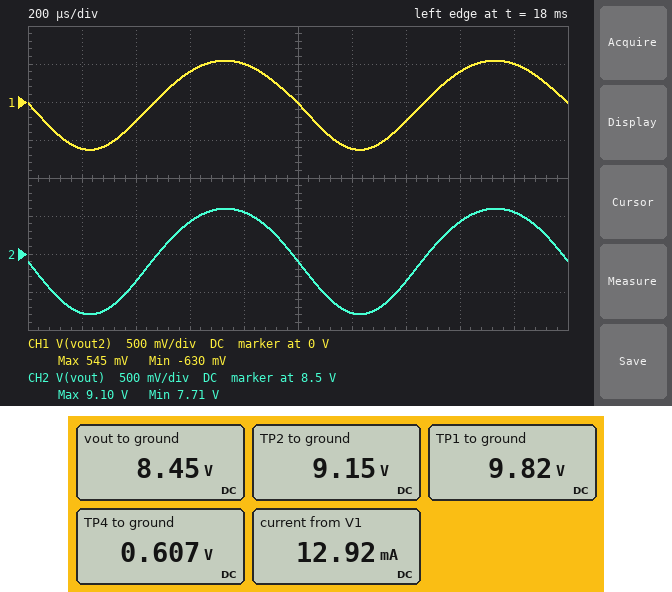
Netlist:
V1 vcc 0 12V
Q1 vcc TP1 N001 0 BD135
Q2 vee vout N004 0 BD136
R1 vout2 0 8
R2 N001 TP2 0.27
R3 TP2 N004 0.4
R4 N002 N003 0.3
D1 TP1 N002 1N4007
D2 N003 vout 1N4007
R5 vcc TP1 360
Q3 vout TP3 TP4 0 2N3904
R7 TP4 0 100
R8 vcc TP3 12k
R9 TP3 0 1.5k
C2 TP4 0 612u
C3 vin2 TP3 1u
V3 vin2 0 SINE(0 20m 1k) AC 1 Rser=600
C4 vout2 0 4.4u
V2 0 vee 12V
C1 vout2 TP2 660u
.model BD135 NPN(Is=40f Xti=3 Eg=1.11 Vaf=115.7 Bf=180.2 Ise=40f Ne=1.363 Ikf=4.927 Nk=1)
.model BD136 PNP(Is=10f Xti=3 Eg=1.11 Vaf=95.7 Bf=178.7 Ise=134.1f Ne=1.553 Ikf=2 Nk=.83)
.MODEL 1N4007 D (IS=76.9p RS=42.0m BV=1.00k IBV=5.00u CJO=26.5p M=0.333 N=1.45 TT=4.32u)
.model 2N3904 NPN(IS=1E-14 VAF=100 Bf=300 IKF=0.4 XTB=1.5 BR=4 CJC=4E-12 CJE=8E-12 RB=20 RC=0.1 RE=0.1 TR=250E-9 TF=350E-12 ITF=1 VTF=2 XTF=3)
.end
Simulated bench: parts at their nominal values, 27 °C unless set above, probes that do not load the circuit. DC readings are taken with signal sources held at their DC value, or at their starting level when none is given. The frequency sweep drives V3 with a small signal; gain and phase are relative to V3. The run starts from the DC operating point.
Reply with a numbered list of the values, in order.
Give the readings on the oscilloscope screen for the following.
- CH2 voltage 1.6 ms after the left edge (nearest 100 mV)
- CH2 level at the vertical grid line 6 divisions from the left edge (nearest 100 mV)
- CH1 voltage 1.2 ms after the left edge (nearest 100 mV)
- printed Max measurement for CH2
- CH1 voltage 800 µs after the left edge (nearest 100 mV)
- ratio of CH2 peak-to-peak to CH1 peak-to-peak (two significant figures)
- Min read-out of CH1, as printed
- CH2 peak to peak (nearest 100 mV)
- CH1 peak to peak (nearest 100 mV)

1. 8.9 V
2. 7.7 V
3. -600 mV
4. 9.10 V
5. 500 mV
6. 1.2
7. -630 mV
8. 1.4 V
9. 1.2 V
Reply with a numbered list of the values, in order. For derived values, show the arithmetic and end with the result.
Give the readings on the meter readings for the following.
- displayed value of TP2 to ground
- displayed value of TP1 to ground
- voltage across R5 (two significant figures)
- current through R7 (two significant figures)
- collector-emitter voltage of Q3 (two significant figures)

1. 9.15 V
2. 9.82 V
3. 12 V - 9.82 V = 2.2 V
4. (607 mV) / 100 Ω = 6.1 mA
5. 8.45 V - 607 mV = 7.8 V
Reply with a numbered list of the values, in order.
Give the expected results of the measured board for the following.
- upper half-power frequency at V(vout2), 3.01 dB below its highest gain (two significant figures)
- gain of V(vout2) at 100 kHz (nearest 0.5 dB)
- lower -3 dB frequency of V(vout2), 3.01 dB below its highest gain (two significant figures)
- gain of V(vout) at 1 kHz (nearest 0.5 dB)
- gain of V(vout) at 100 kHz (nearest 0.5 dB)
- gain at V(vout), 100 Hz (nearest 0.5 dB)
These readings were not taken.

1. 13 kHz
2. 11.0 dB
3. 150 Hz
4. 31.0 dB
5. 27.0 dB
6. 26.0 dB
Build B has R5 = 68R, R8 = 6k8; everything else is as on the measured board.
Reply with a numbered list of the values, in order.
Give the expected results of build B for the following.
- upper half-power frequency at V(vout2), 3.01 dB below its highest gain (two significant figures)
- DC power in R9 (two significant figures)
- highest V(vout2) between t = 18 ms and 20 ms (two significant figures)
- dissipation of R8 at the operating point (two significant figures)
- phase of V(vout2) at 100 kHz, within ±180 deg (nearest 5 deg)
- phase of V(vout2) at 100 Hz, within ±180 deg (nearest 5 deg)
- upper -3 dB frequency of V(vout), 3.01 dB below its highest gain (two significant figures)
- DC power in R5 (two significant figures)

1. 32 kHz
2. 3.0 mW
3. 220 mV
4. 14 mW
5. 105 deg
6. -85 deg
7. 120 kHz
8. 13 mW
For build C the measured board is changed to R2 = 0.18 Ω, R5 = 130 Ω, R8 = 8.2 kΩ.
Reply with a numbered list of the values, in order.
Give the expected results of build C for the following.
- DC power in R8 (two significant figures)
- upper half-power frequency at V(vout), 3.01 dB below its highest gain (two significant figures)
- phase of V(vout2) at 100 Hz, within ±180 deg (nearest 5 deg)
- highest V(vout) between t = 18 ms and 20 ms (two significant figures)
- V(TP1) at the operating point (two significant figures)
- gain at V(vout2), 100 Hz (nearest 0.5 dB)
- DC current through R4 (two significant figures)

1. 13 mW
2. 53 kHz
3. -90 deg
4. 9.6 V
5. 11 V
6. 18.5 dB
7. 11 mA
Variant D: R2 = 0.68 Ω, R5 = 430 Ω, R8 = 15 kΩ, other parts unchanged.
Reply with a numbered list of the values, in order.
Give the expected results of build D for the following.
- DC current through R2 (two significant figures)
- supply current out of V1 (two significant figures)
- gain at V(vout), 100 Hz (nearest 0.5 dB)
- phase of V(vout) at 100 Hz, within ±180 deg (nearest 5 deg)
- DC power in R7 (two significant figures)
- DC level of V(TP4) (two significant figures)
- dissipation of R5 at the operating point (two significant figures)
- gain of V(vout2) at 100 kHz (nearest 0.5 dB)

1. 3.1 mA
2. 7.7 mA
3. 26.0 dB
4. -120 deg
5. 1.5 mW
6. 390 mV
7. 6.4 mW
8. 5.5 dB
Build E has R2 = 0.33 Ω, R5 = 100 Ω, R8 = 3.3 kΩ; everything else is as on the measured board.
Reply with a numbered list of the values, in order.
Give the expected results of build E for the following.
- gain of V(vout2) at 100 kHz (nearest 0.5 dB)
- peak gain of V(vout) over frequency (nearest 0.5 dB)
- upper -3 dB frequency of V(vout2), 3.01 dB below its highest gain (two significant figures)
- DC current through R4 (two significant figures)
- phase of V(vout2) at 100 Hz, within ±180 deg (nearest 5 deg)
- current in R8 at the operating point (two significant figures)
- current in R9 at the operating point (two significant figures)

1. 18.0 dB
2. 27.5 dB
3. 39 kHz
4. 29 mA
5. -75 deg
6. 2.5 mA
7. 2.4 mA
